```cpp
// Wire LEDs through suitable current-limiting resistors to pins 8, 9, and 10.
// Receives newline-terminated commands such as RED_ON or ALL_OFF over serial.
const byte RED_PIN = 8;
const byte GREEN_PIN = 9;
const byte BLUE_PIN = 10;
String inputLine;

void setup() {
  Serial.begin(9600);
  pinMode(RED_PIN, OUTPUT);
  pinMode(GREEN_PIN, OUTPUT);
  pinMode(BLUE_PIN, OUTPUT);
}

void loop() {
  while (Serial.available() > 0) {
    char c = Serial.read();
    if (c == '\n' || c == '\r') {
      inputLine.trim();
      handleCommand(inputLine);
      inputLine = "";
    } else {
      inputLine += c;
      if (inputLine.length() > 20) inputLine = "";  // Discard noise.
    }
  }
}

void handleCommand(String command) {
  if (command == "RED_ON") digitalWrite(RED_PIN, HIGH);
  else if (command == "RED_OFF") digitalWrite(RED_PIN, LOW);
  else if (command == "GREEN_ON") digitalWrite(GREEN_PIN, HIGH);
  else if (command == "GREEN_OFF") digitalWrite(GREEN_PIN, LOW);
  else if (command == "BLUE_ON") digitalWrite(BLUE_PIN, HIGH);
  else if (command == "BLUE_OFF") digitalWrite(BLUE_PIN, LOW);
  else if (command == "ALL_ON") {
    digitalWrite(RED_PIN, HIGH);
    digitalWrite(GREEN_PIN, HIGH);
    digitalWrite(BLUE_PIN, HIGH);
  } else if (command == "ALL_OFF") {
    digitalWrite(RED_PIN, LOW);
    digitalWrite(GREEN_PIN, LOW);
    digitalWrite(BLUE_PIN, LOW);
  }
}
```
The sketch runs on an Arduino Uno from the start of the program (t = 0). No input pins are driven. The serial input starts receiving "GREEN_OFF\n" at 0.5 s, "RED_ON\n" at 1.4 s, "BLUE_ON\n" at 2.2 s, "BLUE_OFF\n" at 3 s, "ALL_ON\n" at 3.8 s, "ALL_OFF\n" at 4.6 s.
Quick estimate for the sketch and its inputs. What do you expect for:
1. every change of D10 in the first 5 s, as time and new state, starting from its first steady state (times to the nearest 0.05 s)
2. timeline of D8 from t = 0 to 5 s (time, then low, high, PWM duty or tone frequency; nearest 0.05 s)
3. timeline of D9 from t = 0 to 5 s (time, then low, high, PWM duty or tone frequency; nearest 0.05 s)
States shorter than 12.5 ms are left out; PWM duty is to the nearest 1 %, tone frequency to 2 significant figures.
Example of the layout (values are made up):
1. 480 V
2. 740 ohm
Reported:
1. 0 s low; 2.2 s high; 3 s low; 3.8 s high; 4.6 s low
2. 0 s low; 1.4 s high; 4.6 s low
3. 0 s low; 3.8 s high; 4.6 s low
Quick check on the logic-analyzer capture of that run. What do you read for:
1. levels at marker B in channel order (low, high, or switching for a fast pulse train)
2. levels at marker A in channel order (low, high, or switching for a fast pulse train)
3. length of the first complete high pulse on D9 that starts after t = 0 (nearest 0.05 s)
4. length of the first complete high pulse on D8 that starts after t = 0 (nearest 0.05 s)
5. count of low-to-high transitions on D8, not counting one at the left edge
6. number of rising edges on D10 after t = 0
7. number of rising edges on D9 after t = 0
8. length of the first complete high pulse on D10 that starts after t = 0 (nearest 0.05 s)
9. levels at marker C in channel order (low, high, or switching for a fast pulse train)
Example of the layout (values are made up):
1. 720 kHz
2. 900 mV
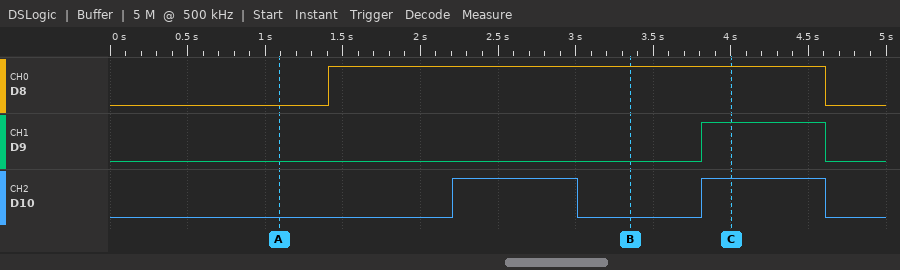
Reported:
1. D8 high, D9 low, D10 low
2. D8 low, D9 low, D10 low
3. 0.80 s
4. 3.20 s
5. 1
6. 2
7. 1
8. 0.80 s
9. D8 high, D9 high, D10 high
